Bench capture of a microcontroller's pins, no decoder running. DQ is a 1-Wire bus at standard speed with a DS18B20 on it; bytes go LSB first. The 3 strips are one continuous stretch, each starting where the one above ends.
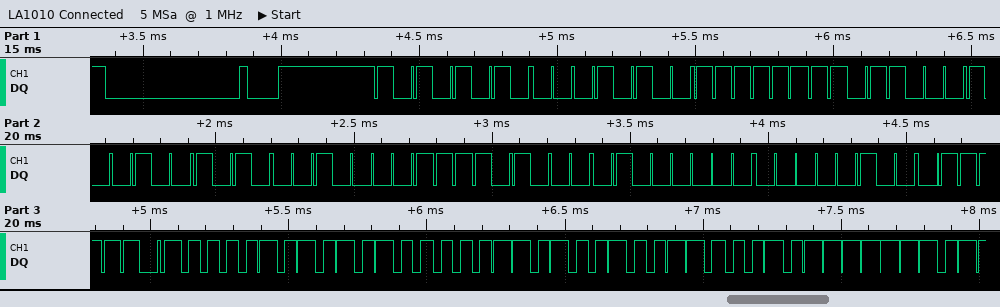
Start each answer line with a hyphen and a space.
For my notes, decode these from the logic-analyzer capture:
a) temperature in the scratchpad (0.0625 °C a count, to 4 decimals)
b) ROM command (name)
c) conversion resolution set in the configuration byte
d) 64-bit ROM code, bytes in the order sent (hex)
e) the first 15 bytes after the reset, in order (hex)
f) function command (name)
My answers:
- 85.0000 °C
- Match ROM
- 12 bits
- 28 FF 46 52 84 17 02 20
- 55 28 FF 46 52 84 17 02 20 BE 50 05 4B 46 7F
- Read Scratchpad
